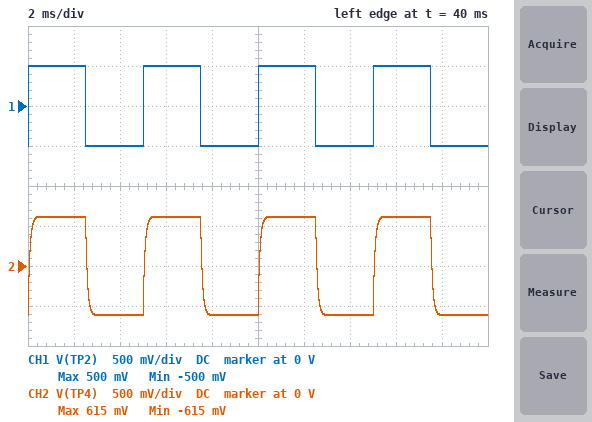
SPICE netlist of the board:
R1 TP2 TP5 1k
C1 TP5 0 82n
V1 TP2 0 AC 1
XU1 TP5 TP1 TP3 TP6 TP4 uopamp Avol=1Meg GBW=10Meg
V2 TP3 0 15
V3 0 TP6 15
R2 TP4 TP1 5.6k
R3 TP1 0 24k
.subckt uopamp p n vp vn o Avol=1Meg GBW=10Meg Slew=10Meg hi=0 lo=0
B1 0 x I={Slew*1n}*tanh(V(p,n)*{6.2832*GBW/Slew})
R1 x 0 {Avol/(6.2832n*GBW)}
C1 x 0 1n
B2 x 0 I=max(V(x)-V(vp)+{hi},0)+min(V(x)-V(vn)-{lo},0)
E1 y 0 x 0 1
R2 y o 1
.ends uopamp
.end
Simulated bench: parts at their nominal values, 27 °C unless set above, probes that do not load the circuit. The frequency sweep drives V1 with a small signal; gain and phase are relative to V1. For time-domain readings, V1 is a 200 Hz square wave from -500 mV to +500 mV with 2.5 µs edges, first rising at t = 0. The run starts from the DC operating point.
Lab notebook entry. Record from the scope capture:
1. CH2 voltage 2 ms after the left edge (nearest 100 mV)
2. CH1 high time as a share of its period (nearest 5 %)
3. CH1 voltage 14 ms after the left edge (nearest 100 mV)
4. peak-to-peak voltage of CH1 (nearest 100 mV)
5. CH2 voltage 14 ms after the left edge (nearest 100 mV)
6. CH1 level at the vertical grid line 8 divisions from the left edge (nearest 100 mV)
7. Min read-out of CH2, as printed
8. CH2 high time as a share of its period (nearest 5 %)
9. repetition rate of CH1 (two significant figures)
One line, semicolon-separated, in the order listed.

600 mV; 50 %; -500 mV; 1.0 V; -600 mV; 500 mV; -615 mV; 50 %; 200 Hz
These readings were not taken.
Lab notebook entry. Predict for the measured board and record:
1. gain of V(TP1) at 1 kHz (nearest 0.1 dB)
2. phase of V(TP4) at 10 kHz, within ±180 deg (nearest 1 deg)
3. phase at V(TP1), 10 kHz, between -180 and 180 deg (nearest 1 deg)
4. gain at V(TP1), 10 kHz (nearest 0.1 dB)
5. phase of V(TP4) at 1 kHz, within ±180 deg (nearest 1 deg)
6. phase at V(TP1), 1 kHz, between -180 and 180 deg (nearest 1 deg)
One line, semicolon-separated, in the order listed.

-1.0 dB; -79 deg; -79 deg; -14.4 dB; -27 deg; -27 deg
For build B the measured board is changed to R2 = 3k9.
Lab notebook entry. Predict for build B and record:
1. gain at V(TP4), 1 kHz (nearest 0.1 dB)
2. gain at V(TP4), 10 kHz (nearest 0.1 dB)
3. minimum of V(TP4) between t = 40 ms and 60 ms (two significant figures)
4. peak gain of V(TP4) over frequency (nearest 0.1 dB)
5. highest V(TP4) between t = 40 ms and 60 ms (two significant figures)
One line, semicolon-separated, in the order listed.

0.3 dB; -13.1 dB; -580 mV; 1.3 dB; 580 mV
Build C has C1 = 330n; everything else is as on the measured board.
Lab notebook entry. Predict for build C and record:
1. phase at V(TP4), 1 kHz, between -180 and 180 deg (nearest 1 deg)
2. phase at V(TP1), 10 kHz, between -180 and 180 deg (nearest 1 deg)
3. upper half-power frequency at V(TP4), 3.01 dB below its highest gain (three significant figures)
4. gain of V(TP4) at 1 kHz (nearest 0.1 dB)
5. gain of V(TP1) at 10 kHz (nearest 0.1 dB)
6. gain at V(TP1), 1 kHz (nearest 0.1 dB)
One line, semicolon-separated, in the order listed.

-64 deg; -87 deg; 482 Hz; -5.4 dB; -26.3 dB; -7.2 dB
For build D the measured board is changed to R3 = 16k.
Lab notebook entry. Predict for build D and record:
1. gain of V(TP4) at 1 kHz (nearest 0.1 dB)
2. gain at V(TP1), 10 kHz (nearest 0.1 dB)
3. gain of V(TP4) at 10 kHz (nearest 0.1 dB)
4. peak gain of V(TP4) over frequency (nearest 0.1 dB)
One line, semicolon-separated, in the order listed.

1.6 dB; -14.4 dB; -11.8 dB; 2.6 dB
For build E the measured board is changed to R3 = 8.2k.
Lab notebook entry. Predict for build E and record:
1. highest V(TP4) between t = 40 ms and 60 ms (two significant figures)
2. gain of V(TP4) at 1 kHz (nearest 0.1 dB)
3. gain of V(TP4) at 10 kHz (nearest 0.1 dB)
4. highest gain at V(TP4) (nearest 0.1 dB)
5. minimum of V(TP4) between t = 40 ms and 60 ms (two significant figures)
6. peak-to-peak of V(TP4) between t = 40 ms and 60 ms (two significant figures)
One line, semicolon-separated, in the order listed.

840 mV; 3.5 dB; -9.9 dB; 4.5 dB; -840 mV; 1.7 V
